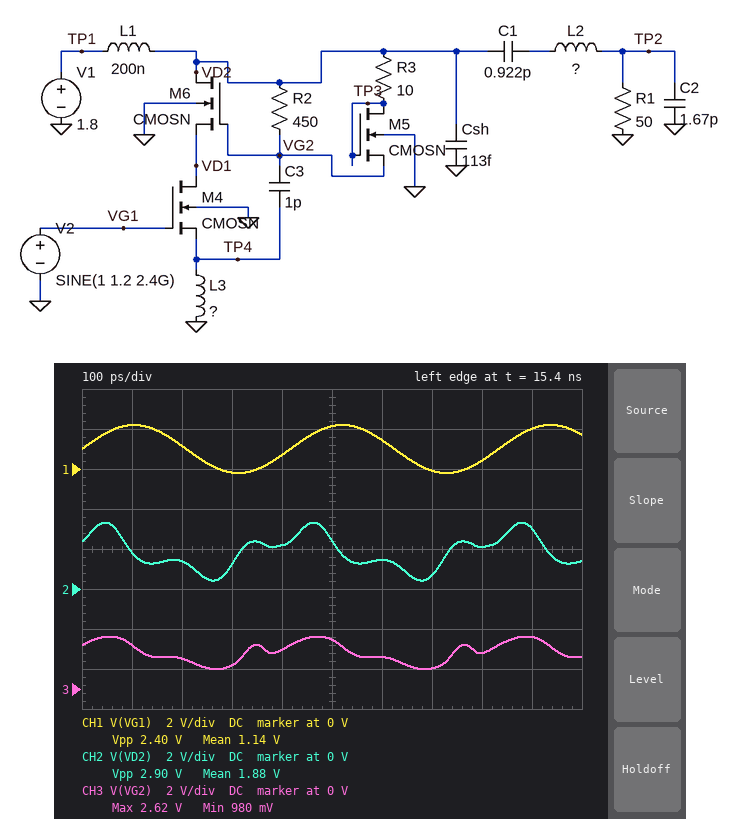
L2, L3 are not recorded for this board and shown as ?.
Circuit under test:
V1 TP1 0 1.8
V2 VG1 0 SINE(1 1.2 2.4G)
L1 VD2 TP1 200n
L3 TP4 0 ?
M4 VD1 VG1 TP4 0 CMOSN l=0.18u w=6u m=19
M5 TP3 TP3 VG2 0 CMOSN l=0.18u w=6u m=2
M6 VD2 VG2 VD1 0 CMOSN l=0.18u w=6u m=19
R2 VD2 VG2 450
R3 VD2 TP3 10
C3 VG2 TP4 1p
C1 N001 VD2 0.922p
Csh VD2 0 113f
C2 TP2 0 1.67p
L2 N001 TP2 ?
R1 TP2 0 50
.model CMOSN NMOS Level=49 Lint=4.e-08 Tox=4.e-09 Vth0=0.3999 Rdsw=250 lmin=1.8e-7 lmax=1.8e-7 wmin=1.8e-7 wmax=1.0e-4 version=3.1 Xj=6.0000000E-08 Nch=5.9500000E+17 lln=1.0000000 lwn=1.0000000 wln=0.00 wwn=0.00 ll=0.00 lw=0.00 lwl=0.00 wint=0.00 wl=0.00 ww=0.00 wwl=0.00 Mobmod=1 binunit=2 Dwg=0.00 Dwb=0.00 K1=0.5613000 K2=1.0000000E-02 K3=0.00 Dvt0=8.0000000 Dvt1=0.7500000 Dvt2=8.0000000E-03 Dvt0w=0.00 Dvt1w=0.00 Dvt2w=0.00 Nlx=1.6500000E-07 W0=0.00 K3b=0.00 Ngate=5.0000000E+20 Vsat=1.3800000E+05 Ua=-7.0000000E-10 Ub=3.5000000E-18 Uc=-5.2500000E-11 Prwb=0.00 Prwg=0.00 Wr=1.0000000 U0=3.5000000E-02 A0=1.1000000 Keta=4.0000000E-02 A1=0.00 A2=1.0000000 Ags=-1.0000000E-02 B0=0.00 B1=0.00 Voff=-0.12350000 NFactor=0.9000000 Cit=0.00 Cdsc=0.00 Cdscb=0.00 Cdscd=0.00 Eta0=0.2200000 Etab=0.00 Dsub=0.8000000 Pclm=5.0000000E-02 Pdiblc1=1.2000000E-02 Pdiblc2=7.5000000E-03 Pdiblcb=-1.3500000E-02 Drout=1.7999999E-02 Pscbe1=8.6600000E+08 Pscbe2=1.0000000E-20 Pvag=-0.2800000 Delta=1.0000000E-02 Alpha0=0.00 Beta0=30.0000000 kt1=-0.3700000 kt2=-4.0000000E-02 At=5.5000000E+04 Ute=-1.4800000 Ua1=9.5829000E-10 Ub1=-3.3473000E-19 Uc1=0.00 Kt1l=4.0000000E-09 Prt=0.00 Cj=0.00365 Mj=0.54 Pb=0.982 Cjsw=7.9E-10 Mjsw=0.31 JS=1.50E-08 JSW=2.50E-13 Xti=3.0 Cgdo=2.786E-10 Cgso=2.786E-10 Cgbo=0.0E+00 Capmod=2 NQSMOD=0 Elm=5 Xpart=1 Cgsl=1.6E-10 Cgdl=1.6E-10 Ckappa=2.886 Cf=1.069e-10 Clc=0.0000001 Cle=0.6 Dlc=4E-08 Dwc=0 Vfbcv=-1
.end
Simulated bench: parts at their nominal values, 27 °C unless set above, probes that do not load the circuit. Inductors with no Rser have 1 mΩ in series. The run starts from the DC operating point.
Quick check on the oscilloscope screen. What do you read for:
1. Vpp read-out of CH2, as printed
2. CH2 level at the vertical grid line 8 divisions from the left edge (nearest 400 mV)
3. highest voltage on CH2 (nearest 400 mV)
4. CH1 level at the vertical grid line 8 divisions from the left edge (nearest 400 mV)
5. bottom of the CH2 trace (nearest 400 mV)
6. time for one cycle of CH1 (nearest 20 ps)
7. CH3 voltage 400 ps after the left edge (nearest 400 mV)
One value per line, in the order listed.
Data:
2.90 V
2.0 V
3.2 V
400 mV
400 mV
420 ps
2.0 V
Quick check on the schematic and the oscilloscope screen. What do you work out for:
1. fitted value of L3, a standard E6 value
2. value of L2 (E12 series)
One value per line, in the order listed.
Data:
1.5 nH
3.9 nH
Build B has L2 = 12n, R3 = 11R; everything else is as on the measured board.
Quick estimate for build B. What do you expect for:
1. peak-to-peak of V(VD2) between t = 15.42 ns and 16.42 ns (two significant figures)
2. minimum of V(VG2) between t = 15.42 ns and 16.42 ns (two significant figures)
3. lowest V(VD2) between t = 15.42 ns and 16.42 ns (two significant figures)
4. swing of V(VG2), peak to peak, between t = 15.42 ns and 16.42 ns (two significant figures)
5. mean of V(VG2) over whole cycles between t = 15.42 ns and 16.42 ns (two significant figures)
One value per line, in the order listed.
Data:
4.7 V
1.4 V
-4.3 mV
1.5 V
2.3 V
